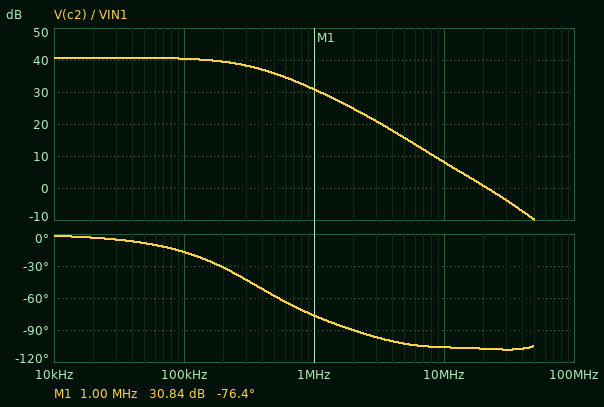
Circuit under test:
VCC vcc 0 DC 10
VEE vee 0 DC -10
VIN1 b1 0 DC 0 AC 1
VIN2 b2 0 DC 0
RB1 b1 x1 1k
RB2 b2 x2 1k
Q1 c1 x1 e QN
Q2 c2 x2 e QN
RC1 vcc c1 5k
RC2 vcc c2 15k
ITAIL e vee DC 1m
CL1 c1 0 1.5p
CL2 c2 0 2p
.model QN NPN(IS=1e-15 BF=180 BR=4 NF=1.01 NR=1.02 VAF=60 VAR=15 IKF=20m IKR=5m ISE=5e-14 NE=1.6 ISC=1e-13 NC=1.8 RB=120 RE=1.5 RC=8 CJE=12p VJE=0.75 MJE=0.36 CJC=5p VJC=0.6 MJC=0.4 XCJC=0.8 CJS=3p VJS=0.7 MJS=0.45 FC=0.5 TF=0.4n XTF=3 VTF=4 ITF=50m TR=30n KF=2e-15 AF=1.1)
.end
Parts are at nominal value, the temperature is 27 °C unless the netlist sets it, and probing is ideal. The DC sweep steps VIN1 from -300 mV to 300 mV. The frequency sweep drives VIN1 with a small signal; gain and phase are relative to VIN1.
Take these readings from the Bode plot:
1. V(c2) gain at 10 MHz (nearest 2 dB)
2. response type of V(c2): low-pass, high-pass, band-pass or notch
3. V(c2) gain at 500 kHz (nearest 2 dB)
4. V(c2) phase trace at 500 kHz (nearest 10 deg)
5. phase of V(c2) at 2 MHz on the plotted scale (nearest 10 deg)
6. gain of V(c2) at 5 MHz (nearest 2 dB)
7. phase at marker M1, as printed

8 dB
low-pass
36 dB
-60 deg
-90 deg
16 dB
-76.4 deg
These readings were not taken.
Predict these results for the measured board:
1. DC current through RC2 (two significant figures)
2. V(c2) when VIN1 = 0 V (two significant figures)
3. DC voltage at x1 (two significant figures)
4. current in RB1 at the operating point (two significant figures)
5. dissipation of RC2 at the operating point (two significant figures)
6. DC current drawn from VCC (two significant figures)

480 µA
2.8 V
-3.9 mV
3.9 µA
3.4 mW
990 µA
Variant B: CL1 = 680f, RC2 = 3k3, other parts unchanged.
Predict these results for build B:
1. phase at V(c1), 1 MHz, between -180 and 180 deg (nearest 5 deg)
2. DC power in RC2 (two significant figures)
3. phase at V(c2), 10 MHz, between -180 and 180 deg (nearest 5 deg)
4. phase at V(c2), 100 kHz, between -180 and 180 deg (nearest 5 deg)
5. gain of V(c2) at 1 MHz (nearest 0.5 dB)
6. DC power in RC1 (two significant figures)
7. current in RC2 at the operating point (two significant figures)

135 deg
820 µW
-90 deg
-5 deg
25.0 dB
1.2 mW
500 µA
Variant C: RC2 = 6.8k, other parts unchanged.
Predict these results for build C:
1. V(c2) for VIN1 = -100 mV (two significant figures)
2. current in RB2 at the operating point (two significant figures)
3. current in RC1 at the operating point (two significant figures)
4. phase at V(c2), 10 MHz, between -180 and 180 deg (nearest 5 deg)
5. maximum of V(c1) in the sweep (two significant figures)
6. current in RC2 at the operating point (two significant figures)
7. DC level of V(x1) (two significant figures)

3.5 V
3.8 µA
500 µA
-100 deg
10 V
490 µA
-3.8 mV
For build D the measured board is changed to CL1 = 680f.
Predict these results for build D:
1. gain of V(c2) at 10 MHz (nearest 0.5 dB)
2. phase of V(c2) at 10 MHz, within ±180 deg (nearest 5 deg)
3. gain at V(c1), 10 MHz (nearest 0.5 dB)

7.5 dB
-110 deg
10.0 dB
